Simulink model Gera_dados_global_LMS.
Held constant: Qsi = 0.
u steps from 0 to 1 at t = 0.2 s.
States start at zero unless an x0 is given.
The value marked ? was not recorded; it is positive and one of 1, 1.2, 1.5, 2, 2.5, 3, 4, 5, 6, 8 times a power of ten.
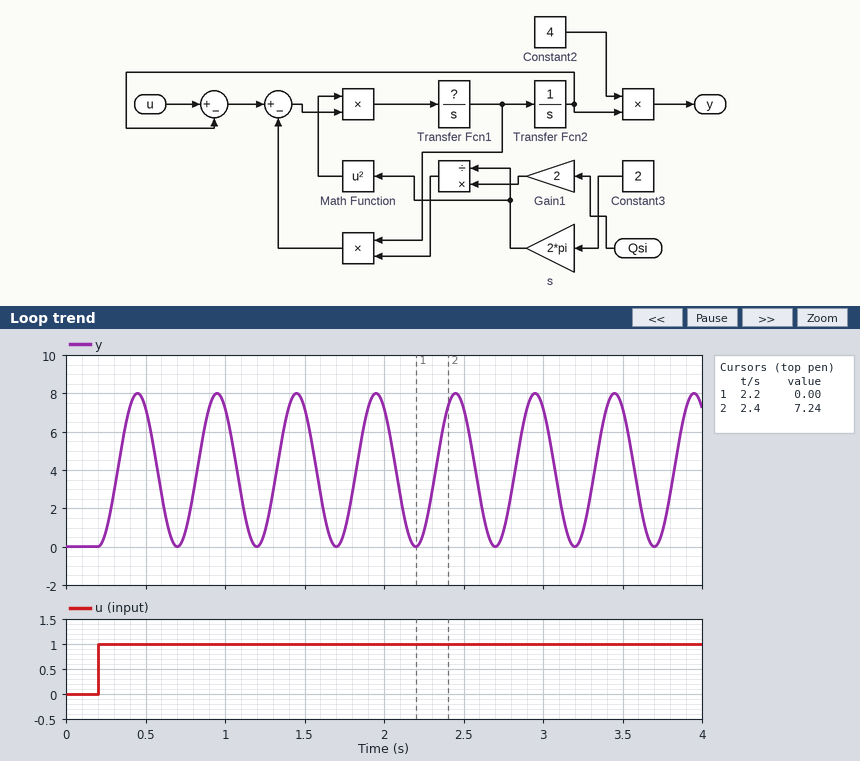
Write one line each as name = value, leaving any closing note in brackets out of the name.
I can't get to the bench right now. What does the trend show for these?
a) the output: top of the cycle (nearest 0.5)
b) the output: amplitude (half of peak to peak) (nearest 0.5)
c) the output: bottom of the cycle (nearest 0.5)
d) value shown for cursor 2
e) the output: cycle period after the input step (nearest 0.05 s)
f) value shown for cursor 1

the output: top of the cycle = 8.0
the output: amplitude (half of peak to peak) = 4.0
the output: bottom of the cycle = 0.0
value shown for cursor 2 = 7.24
the output: cycle period after the input step = 0.50 s
value shown for cursor 1 = 0.00
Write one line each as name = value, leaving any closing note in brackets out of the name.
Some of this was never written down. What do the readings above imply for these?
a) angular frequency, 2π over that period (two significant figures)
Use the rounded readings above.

angular frequency, 2π over that period = 13 rad/s
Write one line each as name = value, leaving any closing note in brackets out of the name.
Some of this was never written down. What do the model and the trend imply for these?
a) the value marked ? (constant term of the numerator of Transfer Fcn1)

the value marked ? = 1
